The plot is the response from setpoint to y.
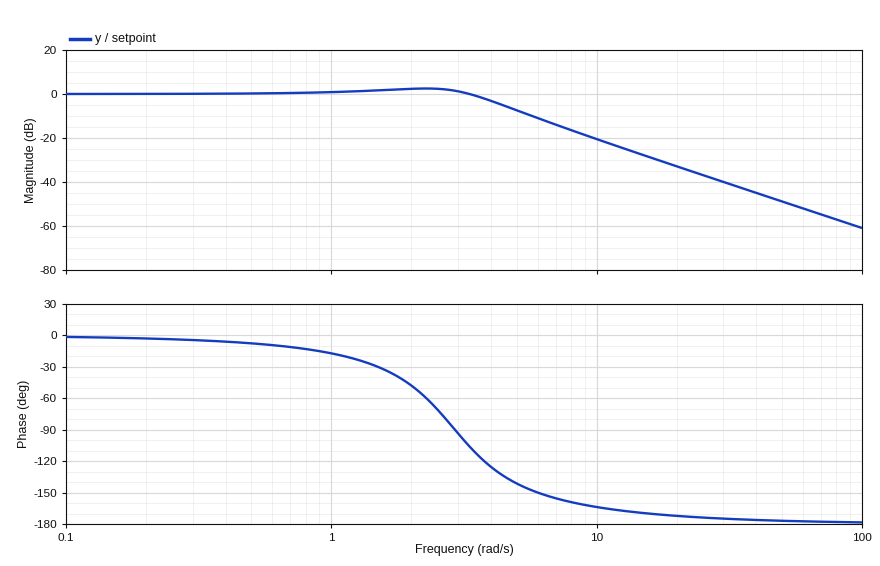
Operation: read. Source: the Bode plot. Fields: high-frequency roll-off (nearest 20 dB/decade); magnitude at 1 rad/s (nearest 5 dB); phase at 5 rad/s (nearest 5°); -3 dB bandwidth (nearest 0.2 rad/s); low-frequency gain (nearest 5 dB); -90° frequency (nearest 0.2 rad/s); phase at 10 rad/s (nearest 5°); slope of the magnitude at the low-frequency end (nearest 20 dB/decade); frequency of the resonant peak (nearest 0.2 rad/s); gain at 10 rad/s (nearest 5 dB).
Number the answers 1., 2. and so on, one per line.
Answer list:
1. -40 dB/decade
2. 0 dB
3. -140°
4. 4.0 rad/s
5. 0 dB
6. 3.0 rad/s
7. -165°
8. 0 dB/decade
9. 2.2 rad/s
10. -20 dB
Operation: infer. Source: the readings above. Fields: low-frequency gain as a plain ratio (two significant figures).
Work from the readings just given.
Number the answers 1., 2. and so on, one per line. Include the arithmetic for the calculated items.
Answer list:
1. 10^(0 / 20) = 1.0
